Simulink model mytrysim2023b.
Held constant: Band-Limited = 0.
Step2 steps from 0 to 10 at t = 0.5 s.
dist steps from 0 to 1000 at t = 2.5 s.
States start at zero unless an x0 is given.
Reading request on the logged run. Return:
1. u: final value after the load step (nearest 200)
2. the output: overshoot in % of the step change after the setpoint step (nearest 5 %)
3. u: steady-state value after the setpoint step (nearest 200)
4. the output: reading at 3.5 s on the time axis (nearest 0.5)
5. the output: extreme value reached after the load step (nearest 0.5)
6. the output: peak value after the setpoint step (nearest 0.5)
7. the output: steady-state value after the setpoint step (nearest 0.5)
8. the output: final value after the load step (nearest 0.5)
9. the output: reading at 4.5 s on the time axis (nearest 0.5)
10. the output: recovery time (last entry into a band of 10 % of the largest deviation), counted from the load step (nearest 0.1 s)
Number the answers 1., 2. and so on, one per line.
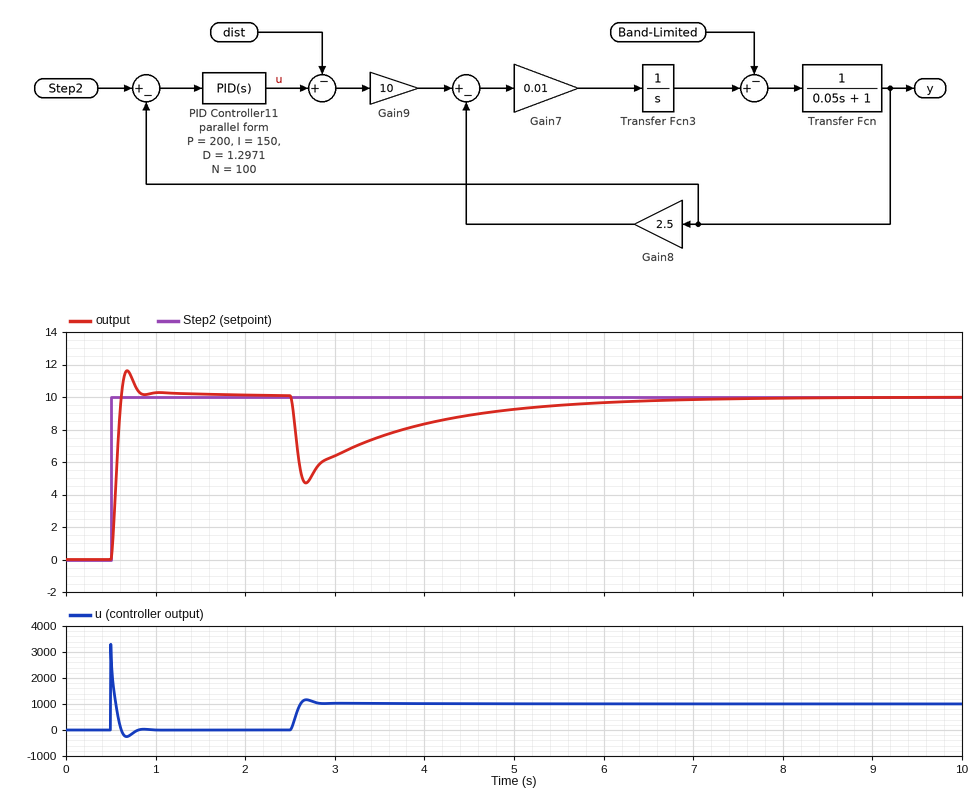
1. 1000
2. 15 %
3. 0
4. 7.5
5. 4.5
6. 11.5
7. 10.0
8. 10.0
9. 9.0
10. 2.9 s
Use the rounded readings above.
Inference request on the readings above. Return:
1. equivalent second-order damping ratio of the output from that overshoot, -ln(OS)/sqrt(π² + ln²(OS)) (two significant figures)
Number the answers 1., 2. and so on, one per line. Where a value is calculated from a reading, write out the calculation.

1. ln(0.15) = -1.897; 1.897 / sqrt(9.870 + 3.599) = 0.52
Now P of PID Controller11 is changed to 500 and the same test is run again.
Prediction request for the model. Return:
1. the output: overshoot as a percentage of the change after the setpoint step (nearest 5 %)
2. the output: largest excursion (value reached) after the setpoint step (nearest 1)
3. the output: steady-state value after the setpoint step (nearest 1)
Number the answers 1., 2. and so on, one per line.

1. 30 %
2. 13
3. 10
